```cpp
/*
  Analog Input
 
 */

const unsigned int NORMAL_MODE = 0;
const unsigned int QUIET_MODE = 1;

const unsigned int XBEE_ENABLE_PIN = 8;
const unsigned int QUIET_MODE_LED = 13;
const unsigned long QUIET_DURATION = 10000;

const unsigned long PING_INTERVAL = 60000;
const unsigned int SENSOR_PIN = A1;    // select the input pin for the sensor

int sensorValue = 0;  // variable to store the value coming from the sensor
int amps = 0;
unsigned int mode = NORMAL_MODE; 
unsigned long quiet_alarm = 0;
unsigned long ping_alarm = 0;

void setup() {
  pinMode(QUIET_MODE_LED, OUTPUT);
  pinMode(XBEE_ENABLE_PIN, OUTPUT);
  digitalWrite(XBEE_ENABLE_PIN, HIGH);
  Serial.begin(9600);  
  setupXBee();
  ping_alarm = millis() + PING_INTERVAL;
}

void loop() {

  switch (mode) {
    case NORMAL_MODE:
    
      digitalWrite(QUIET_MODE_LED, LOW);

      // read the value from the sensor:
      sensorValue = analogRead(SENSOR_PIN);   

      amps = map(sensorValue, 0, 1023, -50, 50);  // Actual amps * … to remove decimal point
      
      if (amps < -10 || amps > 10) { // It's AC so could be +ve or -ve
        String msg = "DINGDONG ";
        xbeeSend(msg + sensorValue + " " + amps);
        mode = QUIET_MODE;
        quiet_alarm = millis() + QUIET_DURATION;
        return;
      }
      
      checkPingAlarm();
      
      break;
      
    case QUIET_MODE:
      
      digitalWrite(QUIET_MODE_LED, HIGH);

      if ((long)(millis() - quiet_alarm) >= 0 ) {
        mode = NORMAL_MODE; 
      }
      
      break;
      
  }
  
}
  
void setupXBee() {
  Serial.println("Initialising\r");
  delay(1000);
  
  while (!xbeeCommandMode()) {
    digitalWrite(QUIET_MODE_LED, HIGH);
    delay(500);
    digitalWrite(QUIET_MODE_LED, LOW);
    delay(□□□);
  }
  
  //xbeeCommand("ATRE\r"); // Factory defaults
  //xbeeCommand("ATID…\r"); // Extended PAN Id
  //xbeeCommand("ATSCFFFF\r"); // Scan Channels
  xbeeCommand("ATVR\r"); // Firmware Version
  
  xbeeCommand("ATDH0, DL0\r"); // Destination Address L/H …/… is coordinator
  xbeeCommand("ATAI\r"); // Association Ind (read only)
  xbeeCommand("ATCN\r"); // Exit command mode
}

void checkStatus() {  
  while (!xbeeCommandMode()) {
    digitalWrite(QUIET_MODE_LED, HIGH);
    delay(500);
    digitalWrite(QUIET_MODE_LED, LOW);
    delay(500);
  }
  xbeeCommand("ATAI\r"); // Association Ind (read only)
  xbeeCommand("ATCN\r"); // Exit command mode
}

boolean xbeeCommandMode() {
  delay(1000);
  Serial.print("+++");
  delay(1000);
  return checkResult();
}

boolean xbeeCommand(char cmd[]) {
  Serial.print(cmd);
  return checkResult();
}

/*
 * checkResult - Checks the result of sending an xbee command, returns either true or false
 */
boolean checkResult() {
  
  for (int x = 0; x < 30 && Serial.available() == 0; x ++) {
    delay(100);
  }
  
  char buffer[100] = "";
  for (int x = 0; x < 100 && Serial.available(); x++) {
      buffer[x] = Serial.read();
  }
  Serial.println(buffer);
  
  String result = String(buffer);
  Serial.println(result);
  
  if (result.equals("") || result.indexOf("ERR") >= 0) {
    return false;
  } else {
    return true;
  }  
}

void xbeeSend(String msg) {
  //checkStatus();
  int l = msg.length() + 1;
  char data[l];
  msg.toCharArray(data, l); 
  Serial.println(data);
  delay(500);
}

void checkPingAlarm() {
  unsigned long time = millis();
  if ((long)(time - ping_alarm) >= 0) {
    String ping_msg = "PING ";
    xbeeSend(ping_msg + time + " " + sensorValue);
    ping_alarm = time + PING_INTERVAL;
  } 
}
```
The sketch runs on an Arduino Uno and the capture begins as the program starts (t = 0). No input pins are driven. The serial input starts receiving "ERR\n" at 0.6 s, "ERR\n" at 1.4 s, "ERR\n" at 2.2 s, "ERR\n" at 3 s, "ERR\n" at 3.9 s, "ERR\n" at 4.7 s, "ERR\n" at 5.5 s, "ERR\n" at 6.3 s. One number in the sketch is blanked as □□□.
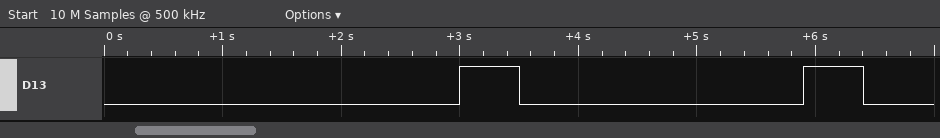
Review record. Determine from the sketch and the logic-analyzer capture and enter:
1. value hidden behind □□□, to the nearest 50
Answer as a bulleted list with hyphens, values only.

- 400
